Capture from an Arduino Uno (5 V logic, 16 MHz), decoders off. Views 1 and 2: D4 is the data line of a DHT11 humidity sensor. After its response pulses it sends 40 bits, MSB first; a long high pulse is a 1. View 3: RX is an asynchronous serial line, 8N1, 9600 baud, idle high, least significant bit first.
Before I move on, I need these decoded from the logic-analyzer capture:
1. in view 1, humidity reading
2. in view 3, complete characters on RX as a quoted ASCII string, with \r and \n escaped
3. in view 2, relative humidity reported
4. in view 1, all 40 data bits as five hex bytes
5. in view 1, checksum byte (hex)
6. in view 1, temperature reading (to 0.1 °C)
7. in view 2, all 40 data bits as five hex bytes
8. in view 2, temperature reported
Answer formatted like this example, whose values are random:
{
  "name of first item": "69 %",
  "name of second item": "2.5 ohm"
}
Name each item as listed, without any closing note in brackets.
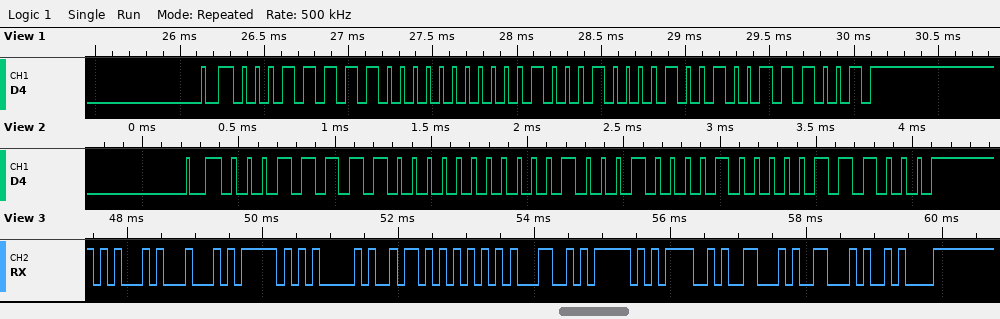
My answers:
{
  "in view 1, humidity reading": "31 %",
  "in view 3, complete characters on RX as a quoted ASCII string, with \\r and \\n escaped": "\"ED_AZUL_OFF\\n\"",
  "in view 2, relative humidity reported": "31 %",
  "in view 1, all 40 data bits as five hex bytes": "1F 00 11 09 39",
  "in view 1, checksum byte": "0x39",
  "in view 1, temperature reading": "17.9 °C",
  "in view 2, all 40 data bits as five hex bytes": "1F 00 11 08 38",
  "in view 2, temperature reported": "17.8 °C"
}
